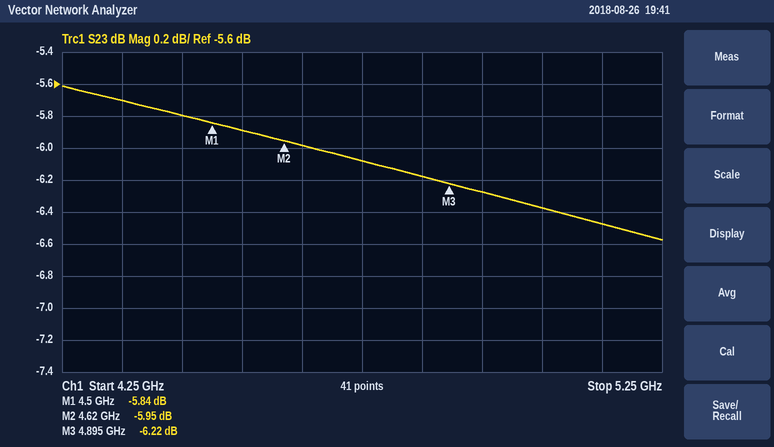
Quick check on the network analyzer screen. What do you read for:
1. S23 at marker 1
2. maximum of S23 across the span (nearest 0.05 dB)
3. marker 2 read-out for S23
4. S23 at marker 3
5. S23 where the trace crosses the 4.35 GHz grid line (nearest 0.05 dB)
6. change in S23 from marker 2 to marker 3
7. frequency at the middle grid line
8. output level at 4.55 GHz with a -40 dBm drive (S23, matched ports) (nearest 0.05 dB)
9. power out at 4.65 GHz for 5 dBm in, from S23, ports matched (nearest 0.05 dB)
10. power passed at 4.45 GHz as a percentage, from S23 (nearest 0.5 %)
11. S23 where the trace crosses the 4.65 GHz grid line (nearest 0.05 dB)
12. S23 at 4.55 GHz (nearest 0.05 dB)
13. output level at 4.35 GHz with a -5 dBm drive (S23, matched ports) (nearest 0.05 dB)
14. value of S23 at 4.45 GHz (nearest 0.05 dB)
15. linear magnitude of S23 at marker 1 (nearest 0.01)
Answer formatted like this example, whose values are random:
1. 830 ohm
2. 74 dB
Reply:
1. -5.84 dB
2. -5.60 dB
3. -5.95 dB
4. -6.22 dB
5. -5.70 dB
6. -0.27 dB
7. 4.75 GHz
8. -45.90 dBm
9. -1.00 dBm
10. 26.5 %
11. -6.00 dB
12. -5.90 dB
13. -10.70 dBm
14. -5.80 dB
15. 0.51
